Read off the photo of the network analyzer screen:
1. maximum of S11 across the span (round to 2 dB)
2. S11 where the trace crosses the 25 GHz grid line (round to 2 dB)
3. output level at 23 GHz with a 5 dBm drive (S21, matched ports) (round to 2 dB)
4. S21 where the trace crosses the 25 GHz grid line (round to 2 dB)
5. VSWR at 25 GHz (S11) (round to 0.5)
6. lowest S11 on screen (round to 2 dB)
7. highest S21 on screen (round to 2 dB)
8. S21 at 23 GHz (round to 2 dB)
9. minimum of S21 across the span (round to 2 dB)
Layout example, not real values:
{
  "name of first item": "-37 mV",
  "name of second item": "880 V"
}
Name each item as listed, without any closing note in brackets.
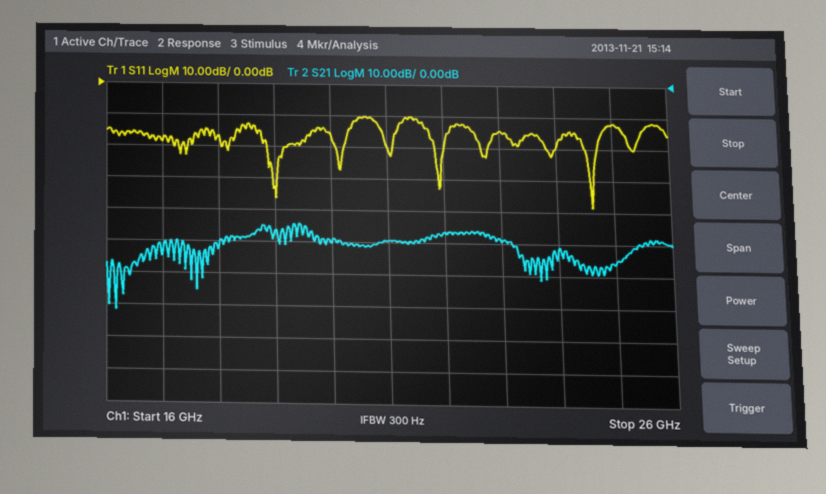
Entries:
{
  "maximum of S11 across the span": "-10 dB",
  "S11 where the trace crosses the 25 GHz grid line": "-12 dB",
  "output level at 23 GHz with a 5 dBm drive (S21, matched ports)": "-44 dBm",
  "S21 where the trace crosses the 25 GHz grid line": "-56 dB",
  "VSWR at 25 GHz (S11)": "1.5",
  "lowest S11 on screen": "-38 dB",
  "highest S21 on screen": "-44 dB",
  "S21 at 23 GHz": "-50 dB",
  "minimum of S21 across the span": "-72 dB"
}
